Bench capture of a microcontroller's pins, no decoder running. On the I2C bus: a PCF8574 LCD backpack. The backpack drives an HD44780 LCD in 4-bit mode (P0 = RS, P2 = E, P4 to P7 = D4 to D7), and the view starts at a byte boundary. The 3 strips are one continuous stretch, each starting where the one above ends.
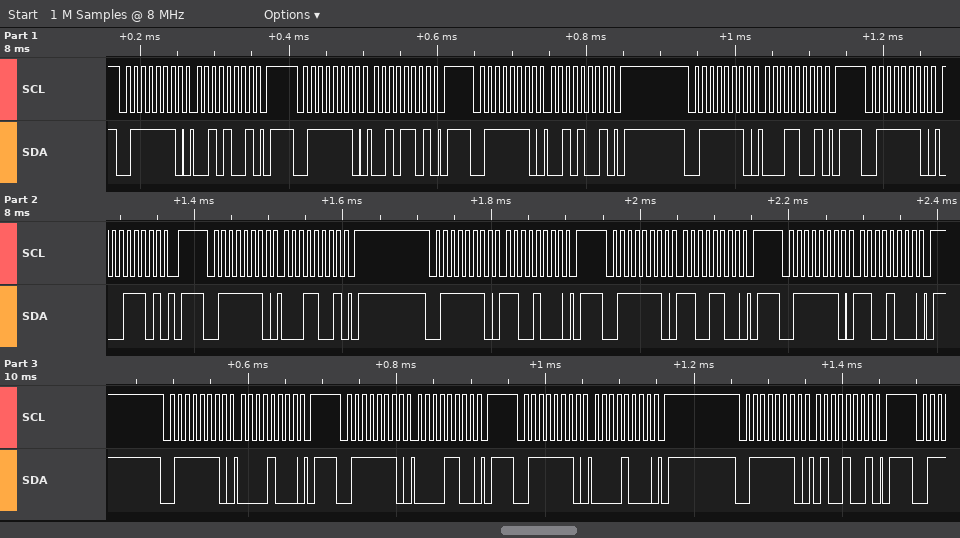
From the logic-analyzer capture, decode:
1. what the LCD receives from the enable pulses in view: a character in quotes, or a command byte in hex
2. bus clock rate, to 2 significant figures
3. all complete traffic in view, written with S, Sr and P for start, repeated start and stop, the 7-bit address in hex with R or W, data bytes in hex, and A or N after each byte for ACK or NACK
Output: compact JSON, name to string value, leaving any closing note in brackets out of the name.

{"what the LCD receives from the enable pulses in view: a character in quotes, or a command byte in hex": "'!' 0xC0", "bus clock rate, to 2 significant figures": "100 kHz", "all complete traffic in view, written with S, Sr and P for start, repeated start and stop, the 7-bit address in hex with R or W, data bytes in hex, and A or N after each byte for ACK or NACK": "S 3FW A 29 A P S 3FW A 2D A P S 3FW A 29 A P S 3FW A 19 A P S 3FW A 1D A P S 3FW A 19 A P S 3FW A C8 A P S 3FW A CC A P S 3FW A C8 A P S 3FW A 08 A P S 3FW A 0C A P S 3FW A 08 A P S 3FW A 49 A P"}
